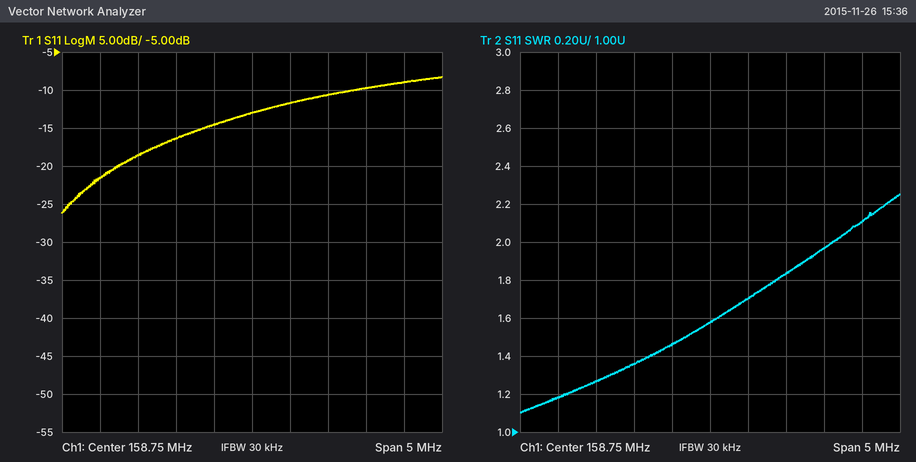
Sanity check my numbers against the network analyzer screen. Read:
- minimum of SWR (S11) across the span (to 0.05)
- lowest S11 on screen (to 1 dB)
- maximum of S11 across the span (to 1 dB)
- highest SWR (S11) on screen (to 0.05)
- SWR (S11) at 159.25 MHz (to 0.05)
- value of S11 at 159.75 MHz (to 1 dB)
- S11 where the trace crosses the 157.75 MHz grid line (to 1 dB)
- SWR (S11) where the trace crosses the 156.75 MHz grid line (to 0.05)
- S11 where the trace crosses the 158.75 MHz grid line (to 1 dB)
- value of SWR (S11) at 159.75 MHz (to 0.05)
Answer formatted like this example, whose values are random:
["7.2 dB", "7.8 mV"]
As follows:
["1.10", "-26 dB", "-8 dB", "2.25", "1.70", "-11 dB", "-16 dB", "1.20", "-13 dB", "1.85"]
